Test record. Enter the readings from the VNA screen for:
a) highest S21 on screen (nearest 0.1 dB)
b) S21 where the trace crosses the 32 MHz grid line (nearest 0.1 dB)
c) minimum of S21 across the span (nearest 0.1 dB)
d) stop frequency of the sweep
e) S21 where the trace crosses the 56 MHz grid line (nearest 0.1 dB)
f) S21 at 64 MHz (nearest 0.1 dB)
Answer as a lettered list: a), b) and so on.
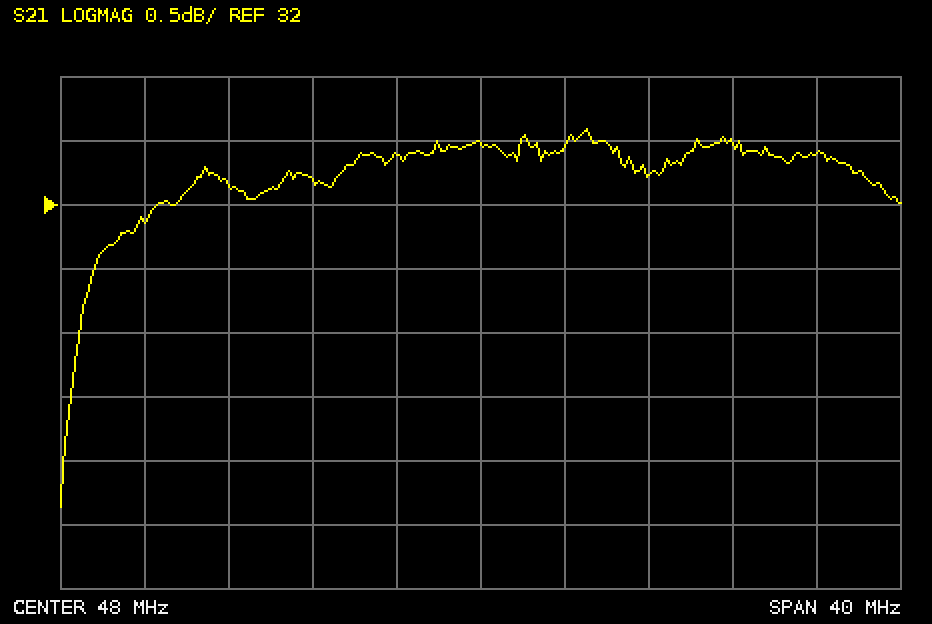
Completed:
a) 32.6 dB
b) 31.9 dB
c) 29.6 dB
d) 68 MHz
e) 32.2 dB
f) 32.4 dB
